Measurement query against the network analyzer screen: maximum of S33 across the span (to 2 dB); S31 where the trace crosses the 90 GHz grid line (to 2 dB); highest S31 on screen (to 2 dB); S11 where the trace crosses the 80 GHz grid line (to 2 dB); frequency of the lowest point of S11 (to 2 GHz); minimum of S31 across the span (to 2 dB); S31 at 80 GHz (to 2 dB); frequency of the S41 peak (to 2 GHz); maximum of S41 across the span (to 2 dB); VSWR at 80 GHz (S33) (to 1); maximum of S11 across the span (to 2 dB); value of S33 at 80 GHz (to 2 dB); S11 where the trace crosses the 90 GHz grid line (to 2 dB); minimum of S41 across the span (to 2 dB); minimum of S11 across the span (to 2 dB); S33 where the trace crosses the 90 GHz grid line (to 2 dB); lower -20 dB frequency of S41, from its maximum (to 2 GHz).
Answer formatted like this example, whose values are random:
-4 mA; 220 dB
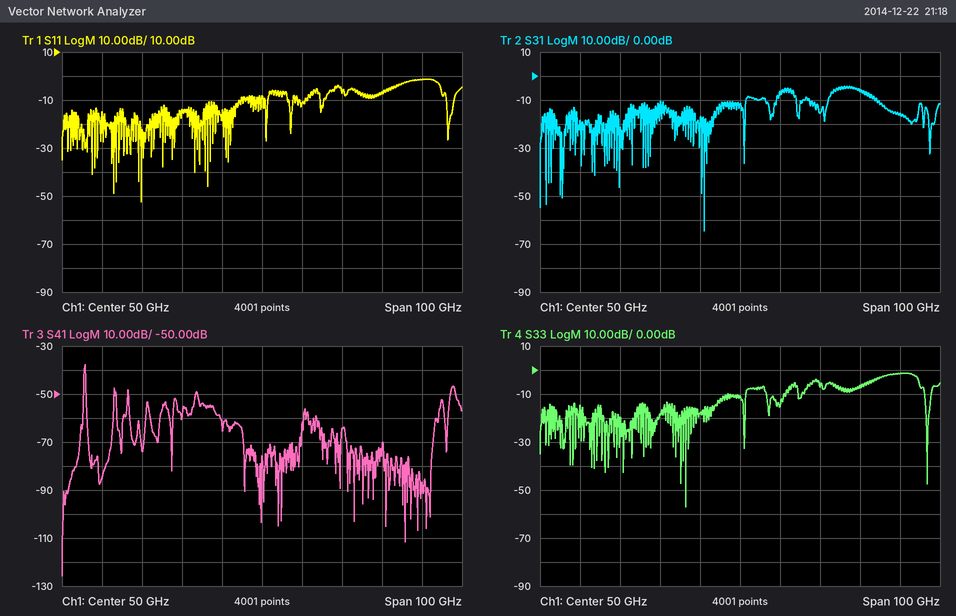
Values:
-2 dB; -16 dB; -4 dB; -6 dB; 20 GHz; -64 dB; -6 dB; 6 GHz; -38 dB; 3; -2 dB; -6 dB; -2 dB; -126 dB; -52 dB; -2 dB; 6 GHz
